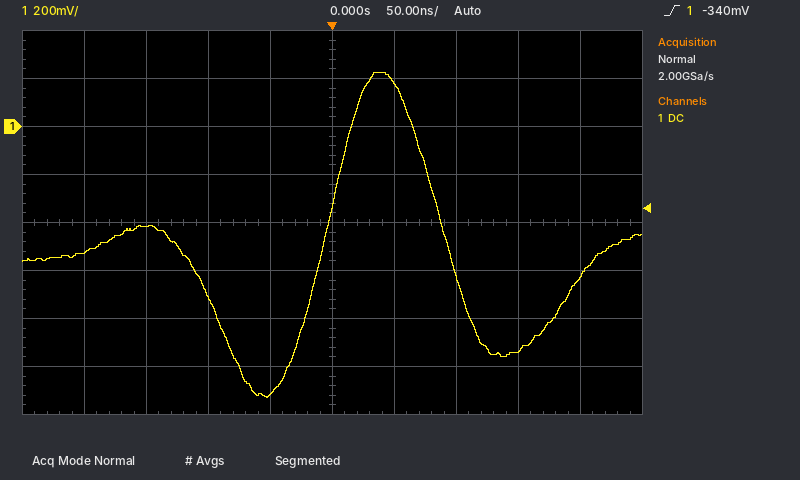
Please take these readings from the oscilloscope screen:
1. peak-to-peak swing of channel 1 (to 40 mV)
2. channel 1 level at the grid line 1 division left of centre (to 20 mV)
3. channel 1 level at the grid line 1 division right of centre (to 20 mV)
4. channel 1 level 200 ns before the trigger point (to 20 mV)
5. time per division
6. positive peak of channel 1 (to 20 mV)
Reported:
1.36 V
-1.12 V
180 mV
-520 mV
50 ns
220 mV
